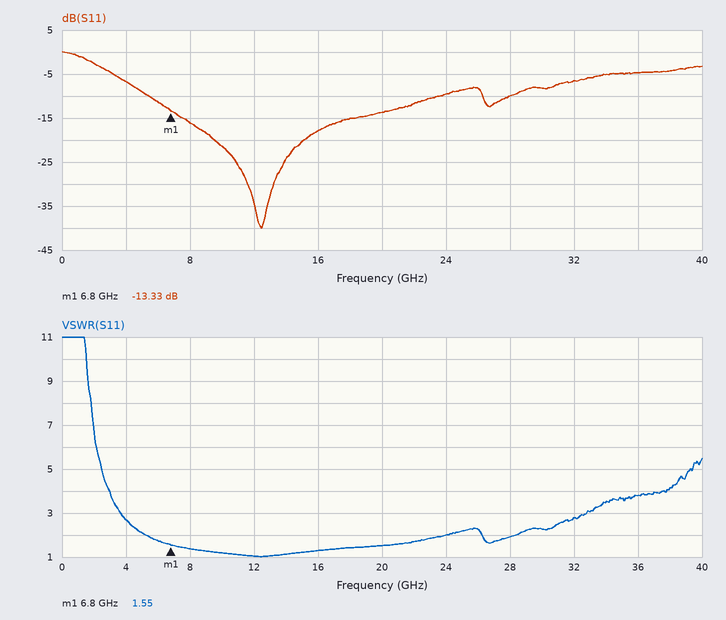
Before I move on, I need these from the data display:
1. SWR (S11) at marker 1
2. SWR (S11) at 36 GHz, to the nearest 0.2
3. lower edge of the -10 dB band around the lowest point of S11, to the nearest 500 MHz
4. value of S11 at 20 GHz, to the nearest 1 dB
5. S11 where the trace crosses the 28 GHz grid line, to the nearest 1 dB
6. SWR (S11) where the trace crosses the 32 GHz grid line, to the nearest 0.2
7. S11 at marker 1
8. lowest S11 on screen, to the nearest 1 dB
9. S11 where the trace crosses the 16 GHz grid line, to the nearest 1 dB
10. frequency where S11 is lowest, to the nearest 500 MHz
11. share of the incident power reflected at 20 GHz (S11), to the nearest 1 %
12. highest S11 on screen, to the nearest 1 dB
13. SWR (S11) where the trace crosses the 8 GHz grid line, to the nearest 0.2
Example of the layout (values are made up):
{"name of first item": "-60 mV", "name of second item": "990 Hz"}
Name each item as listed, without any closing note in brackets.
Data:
{"SWR (S11) at marker 1": "1.55", "SWR (S11) at 36 GHz, to the nearest 0.2": "3.8", "lower edge of the -10 dB band around the lowest point of S11, to the nearest 500 MHz": "5.5 GHz", "value of S11 at 20 GHz, to the nearest 1 dB": "-14 dB", "S11 where the trace crosses the 28 GHz grid line, to the nearest 1 dB": "-10 dB", "SWR (S11) where the trace crosses the 32 GHz grid line, to the nearest 0.2": "2.8", "S11 at marker 1": "-13.33 dB", "lowest S11 on screen, to the nearest 1 dB": "-40 dB", "S11 where the trace crosses the 16 GHz grid line, to the nearest 1 dB": "-18 dB", "frequency where S11 is lowest, to the nearest 500 MHz": "12.5 GHz", "share of the incident power reflected at 20 GHz (S11), to the nearest 1 %": "4 %", "highest S11 on screen, to the nearest 1 dB": "0 dB", "SWR (S11) where the trace crosses the 8 GHz grid line, to the nearest 0.2": "1.4"}
